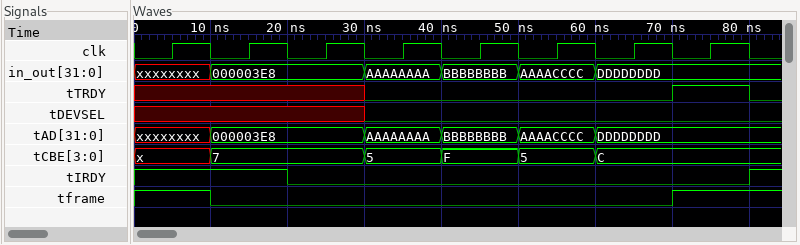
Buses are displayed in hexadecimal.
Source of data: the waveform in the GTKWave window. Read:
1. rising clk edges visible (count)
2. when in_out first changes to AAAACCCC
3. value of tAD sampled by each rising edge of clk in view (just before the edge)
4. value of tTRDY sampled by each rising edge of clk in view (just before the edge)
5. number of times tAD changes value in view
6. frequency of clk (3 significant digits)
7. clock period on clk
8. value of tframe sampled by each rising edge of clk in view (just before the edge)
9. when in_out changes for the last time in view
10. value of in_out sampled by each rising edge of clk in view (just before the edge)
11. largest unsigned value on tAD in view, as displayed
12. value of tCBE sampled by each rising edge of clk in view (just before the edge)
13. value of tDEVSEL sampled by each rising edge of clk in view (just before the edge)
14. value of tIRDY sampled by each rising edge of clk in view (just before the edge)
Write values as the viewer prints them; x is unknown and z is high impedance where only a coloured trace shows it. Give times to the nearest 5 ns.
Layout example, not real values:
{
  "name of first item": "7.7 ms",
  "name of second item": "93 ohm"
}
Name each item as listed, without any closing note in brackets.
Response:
{
  "rising clk edges visible": "8",
  "when in_out first changes to AAAACCCC": "50 ns",
  "value of tAD sampled by each rising edge of clk in view": "xxxxxxxx, 000003E8, 000003E8, AAAAAAAA, BBBBBBBB, AAAACCCC, DDDDDDDD, DDDDDDDD",
  "value of tTRDY sampled by each rising edge of clk in view": "x x x 0 0 0 0 1",
  "number of times tAD changes value in view": "5",
  "frequency of clk": "100 MHz",
  "clock period on clk": "10 ns",
  "value of tframe sampled by each rising edge of clk in view": "1 0 0 0 0 0 0 1",
  "when in_out changes for the last time in view": "60 ns",
  "value of in_out sampled by each rising edge of clk in view": "xxxxxxxx, 000003E8, 000003E8, AAAAAAAA, BBBBBBBB, AAAACCCC, DDDDDDDD, DDDDDDDD",
  "largest unsigned value on tAD in view, as displayed": "DDDDDDDD",
  "value of tCBE sampled by each rising edge of clk in view": "x, 7, 7, 5, F, 5, C, C",
  "value of tDEVSEL sampled by each rising edge of clk in view": "x x x 0 0 0 0 0",
  "value of tIRDY sampled by each rising edge of clk in view": "1 1 0 0 0 0 0 0"
}
